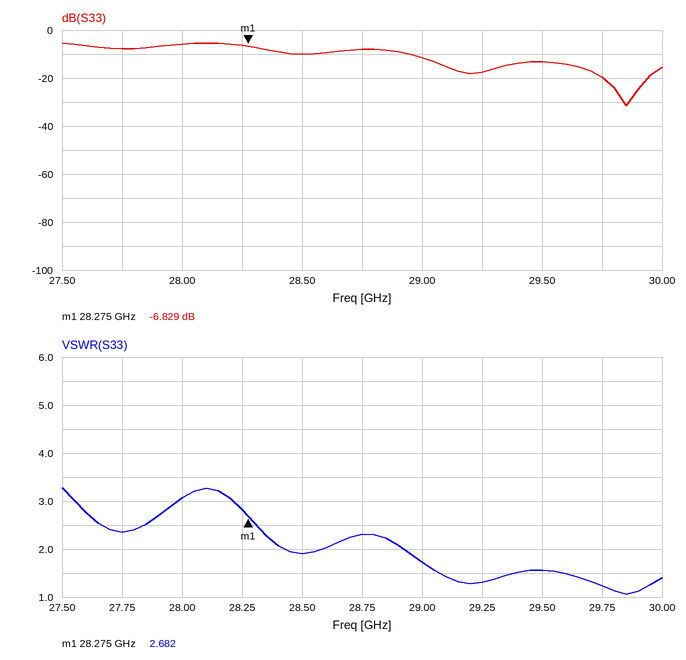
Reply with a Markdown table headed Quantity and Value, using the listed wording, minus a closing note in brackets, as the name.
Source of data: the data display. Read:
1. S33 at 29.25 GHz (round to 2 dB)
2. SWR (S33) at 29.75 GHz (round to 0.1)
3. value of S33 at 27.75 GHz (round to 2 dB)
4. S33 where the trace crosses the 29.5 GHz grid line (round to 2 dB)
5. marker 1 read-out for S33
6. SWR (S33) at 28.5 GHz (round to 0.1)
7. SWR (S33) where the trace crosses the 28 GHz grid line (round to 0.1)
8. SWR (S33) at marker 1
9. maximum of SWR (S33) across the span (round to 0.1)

| Quantity | Value |
|---|---|
| S33 at 29.25 GHz | -18 dB |
| SWR (S33) at 29.75 GHz | 1.2 |
| value of S33 at 27.75 GHz | -8 dB |
| S33 where the trace crosses the 29.5 GHz grid line | -14 dB |
| marker 1 read-out for S33 | -6.829 dB |
| SWR (S33) at 28.5 GHz | 1.9 |
| SWR (S33) where the trace crosses the 28 GHz grid line | 3.1 |
| SWR (S33) at marker 1 | 2.682 |
| maximum of SWR (S33) across the span | 3.3 |
